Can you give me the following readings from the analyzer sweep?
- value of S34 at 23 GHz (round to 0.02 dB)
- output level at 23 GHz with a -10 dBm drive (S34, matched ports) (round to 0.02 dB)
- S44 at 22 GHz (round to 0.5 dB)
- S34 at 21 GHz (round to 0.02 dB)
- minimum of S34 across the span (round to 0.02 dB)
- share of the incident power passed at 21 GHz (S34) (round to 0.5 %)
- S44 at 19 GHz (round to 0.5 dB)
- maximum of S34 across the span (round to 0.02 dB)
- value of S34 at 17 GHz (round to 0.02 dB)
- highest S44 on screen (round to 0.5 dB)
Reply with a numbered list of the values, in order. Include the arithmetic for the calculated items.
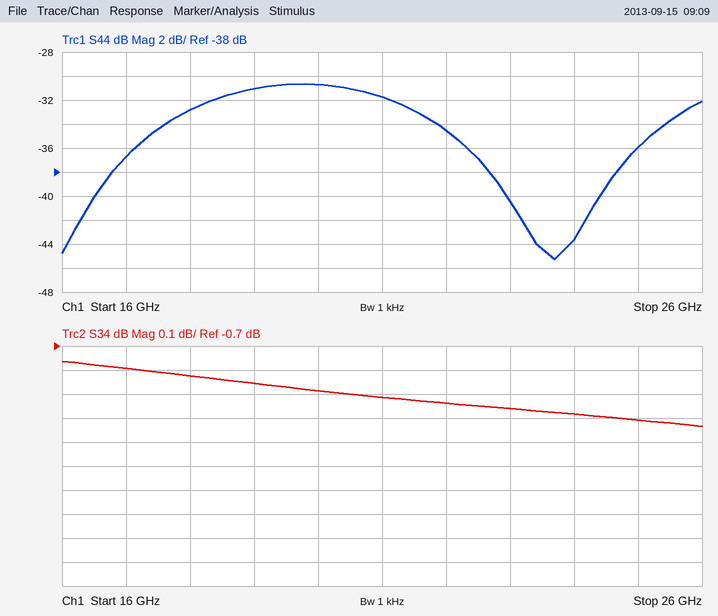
1. -0.96 dB
2. -10 dBm + (-0.96 dB) = -10.96 dBm
3. -34.5 dB
4. -0.92 dB
5. -1.04 dB
6. 10^(-0.92/10) ≈ 80.9 %, so 81.0 % to the nearest 0.5 %
7. -31.0 dB
8. -0.76 dB
9. -0.80 dB
10. -30.5 dB
